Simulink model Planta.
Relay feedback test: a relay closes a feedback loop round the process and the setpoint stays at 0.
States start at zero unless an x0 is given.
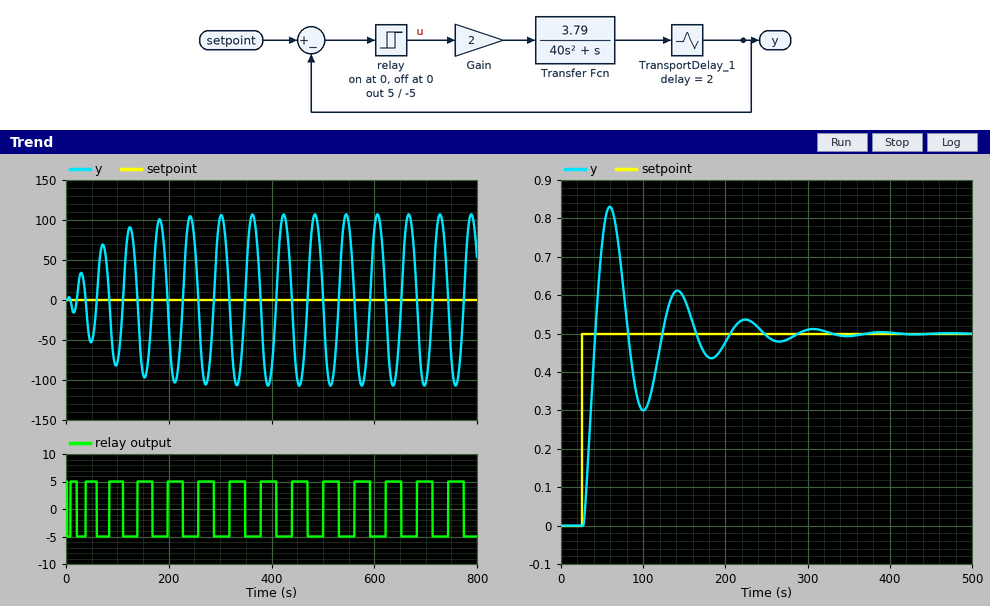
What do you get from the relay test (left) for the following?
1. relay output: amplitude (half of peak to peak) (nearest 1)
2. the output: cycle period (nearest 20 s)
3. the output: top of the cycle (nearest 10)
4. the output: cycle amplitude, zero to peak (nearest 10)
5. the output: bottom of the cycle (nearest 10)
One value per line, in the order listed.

5
60 s
110
110
-110
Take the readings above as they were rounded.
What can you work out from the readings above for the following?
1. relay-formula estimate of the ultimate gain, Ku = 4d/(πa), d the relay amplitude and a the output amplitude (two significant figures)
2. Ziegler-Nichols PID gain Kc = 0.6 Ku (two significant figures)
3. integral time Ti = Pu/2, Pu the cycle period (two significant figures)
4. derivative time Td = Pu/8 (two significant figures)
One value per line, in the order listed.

0.058
0.035
30 s
7.5 s
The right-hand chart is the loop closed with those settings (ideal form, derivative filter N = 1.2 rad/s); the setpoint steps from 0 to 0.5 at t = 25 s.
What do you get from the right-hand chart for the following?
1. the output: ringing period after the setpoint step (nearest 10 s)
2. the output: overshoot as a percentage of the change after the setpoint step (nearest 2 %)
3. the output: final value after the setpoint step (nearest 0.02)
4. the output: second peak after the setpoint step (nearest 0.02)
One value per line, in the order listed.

80 s
66 %
0.50
0.62
